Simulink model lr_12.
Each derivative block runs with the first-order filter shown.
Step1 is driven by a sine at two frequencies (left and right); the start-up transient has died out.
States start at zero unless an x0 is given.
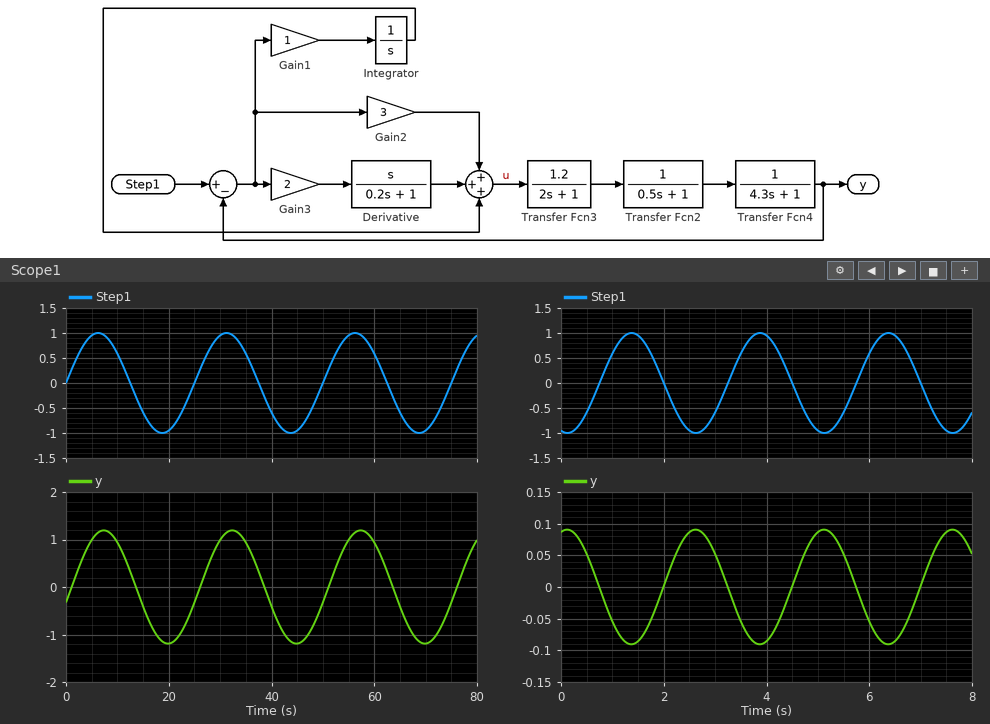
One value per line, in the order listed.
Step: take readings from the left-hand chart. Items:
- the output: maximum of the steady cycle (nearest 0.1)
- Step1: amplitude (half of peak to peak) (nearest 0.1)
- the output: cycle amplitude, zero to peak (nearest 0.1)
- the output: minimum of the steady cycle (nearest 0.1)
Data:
1.2
1.0
1.2
-1.2
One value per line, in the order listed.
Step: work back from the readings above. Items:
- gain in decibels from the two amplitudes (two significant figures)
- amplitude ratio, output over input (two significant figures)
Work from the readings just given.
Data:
1.6 dB
1.2
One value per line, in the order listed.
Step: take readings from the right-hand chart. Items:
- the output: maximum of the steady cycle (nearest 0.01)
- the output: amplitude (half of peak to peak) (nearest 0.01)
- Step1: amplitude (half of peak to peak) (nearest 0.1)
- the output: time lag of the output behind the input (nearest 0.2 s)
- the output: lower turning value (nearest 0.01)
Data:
0.09
0.09
1.0
1.2 s
-0.09
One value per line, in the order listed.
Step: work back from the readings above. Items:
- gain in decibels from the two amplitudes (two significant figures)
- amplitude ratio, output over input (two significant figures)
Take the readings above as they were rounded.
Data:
-21 dB
0.090
